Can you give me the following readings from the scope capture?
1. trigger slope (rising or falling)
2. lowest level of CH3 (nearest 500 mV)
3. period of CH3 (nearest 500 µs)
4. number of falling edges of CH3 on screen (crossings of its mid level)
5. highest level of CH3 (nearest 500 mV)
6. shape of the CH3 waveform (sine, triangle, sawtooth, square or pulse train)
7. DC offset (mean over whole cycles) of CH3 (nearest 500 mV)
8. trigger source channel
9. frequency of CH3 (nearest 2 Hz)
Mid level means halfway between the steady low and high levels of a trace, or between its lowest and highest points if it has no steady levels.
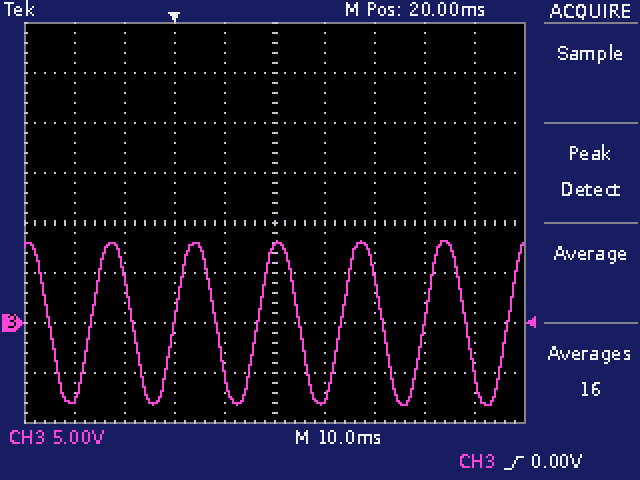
rising
-8.0 V
16.5 ms
6
8.0 V
sine
0.0 V
CH3
60 Hz
